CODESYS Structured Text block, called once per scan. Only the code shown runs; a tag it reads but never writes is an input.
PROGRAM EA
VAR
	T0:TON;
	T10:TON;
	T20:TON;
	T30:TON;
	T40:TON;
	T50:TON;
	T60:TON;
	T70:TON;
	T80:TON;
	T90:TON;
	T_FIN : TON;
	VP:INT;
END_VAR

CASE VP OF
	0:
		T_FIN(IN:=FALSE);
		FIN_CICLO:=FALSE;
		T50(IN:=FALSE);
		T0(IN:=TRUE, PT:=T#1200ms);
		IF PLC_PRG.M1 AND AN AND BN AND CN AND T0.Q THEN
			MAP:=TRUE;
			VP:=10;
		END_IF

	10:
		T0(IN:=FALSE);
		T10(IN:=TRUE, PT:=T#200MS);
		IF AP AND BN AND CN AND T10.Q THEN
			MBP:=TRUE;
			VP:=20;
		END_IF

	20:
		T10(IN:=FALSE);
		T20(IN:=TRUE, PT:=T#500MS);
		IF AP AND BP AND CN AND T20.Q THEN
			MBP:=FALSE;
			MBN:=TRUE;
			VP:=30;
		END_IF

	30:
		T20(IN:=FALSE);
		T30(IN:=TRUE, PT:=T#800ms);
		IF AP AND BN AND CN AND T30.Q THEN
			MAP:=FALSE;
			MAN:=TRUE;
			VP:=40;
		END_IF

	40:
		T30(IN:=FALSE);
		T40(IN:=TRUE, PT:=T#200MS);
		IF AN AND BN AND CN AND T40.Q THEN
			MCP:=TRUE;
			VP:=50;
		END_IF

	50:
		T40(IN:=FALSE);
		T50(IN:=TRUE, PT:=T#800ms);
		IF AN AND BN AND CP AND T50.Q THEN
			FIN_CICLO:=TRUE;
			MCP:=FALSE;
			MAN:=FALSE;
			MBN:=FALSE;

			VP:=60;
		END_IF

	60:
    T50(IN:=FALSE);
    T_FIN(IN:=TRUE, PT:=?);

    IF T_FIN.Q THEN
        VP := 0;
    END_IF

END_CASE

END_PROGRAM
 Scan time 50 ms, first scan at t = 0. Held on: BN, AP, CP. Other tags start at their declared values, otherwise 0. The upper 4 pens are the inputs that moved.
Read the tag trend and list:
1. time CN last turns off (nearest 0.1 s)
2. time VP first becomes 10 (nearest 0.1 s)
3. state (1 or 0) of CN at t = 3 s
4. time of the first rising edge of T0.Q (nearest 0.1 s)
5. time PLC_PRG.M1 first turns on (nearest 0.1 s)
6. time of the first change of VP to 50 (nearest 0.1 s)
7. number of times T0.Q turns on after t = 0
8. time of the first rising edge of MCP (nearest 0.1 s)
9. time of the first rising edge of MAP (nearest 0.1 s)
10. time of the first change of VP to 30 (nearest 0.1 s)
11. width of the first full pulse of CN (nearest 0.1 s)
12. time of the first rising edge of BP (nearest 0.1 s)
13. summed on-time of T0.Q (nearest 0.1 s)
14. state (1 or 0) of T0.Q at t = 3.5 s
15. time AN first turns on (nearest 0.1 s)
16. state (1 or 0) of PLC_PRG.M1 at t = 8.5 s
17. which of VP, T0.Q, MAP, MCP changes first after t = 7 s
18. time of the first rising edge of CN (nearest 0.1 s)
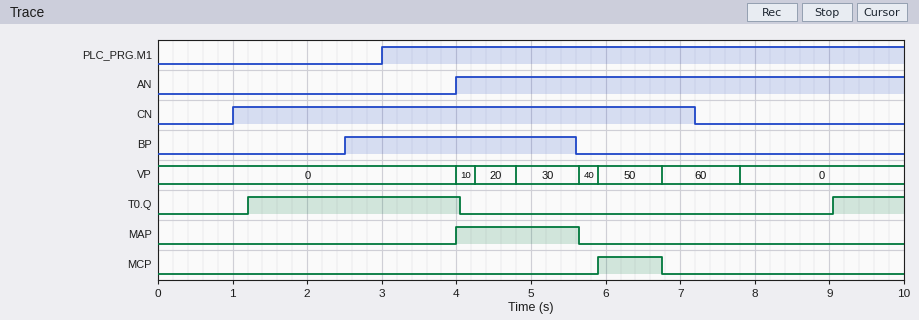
7.2 s
4.0 s
1
1.2 s
3.0 s
5.9 s
2
5.9 s
4.0 s
4.8 s
6.2 s
2.5 s
3.8 s
1
4.0 s
1
VP
1.0 s
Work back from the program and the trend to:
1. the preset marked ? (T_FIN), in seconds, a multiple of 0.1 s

1.0 s
